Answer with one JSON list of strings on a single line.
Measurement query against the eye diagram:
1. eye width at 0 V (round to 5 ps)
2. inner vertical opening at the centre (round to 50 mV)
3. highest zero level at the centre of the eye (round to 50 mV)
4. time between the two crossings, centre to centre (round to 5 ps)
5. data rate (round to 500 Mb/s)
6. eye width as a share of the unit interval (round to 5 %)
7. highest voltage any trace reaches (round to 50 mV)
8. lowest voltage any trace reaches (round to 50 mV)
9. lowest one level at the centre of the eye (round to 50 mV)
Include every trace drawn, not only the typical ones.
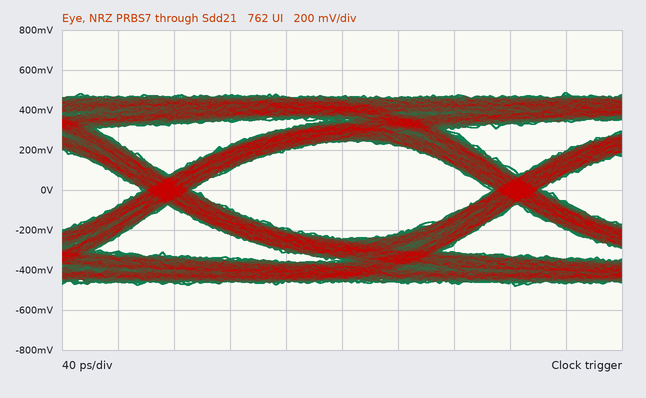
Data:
["215 ps", "500 mV", "-250 mV", "250 ps", "4.0 Gb/s", "85 %", "500 mV", "-500 mV", "250 mV"]
